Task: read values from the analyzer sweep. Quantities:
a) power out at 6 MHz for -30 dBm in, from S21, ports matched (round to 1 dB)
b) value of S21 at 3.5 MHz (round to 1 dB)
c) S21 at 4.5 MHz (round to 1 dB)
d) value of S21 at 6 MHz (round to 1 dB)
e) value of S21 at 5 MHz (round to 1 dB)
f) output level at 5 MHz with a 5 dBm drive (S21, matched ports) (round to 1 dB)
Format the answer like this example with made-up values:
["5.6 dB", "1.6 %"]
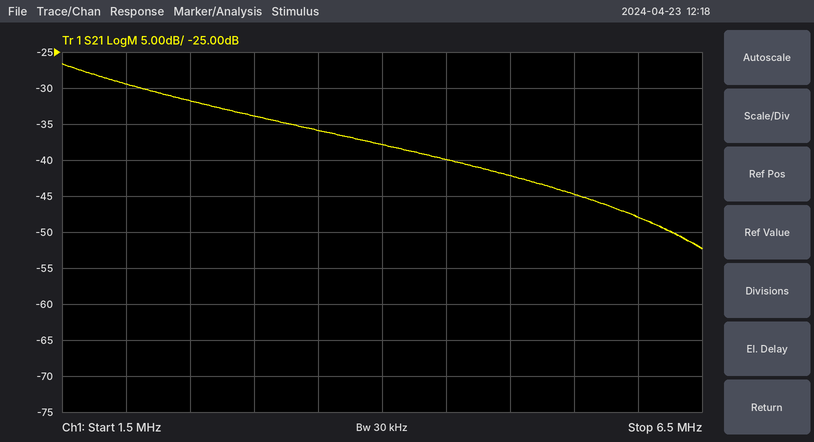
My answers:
["-78 dBm", "-36 dB", "-40 dB", "-48 dB", "-42 dB", "-37 dBm"]
